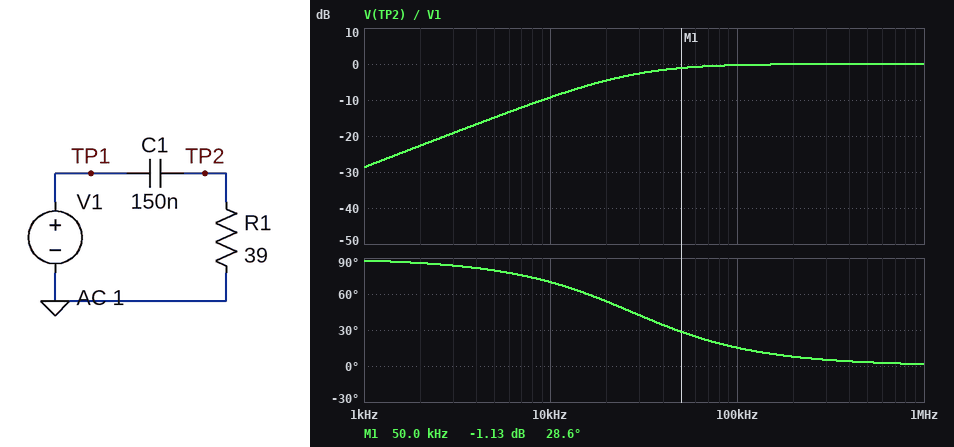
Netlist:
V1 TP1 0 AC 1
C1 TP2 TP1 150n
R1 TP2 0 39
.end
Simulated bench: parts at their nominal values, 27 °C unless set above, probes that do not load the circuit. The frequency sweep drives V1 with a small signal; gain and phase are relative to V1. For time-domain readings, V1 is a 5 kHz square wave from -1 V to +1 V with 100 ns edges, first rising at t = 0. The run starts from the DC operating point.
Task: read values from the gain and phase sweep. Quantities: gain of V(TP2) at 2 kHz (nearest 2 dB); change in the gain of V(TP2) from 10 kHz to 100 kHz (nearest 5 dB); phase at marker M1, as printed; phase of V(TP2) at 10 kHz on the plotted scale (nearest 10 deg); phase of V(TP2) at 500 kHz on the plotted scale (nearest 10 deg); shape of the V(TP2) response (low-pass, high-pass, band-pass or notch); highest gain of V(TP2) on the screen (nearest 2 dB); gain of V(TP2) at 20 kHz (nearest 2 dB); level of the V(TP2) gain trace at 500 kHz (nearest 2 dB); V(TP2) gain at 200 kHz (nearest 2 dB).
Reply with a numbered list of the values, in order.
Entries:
1. -22 dB
2. 10 dB
3. 28.6 deg
4. 70 deg
5. 0 deg
6. high-pass
7. 0 dB
8. -4 dB
9. 0 dB
10. 0 dB
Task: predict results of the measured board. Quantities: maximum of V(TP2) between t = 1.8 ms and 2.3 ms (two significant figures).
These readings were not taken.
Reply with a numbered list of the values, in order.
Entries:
1. 2.0 V
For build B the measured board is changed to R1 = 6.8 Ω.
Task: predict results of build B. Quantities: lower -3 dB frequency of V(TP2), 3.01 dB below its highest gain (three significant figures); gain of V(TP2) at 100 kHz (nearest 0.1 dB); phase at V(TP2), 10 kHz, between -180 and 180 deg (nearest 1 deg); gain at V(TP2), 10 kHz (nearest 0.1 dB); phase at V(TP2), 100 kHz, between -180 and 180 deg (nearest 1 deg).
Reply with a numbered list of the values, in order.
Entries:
1. 156 kHz
2. -5.4 dB
3. 86 deg
4. -23.9 dB
5. 57 deg
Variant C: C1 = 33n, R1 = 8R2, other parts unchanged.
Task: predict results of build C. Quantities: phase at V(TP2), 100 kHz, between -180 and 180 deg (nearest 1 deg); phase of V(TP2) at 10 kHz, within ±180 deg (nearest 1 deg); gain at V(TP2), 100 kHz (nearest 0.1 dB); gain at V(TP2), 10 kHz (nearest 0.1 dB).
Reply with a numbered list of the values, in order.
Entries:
1. 80 deg
2. 89 deg
3. -15.5 dB
4. -35.4 dB
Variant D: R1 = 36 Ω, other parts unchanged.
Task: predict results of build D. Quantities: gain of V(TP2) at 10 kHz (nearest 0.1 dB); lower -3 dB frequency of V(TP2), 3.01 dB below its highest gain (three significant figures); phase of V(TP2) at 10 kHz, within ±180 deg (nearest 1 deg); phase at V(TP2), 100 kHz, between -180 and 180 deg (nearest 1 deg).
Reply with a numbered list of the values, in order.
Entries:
1. -9.9 dB
2. 29.5 kHz
3. 71 deg
4. 16 deg
